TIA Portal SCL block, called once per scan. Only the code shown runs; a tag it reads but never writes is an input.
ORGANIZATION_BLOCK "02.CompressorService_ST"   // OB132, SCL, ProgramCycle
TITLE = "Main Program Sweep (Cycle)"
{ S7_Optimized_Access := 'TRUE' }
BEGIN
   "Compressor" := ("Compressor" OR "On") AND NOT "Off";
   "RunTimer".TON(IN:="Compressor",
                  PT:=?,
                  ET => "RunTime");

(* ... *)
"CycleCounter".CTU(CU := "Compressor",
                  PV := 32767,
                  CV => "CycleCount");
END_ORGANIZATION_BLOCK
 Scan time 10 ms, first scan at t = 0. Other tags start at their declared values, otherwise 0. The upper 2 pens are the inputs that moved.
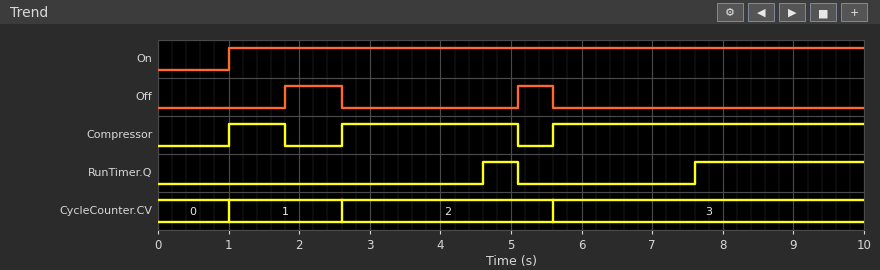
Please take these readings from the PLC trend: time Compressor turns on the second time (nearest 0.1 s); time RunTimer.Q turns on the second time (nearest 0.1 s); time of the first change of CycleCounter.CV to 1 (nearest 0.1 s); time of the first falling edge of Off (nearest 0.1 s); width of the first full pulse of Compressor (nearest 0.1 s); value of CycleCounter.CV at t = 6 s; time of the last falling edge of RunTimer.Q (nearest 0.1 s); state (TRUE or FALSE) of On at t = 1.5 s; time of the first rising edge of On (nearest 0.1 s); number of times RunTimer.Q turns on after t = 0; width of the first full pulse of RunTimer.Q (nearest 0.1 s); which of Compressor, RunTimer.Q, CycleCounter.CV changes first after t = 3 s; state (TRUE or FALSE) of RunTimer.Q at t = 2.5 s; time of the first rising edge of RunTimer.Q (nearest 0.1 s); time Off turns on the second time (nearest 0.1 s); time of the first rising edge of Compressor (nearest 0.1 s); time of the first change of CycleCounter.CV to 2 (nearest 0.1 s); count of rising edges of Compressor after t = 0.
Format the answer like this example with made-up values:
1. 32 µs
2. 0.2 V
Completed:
1. 2.6 s
2. 7.6 s
3. 1.0 s
4. 2.6 s
5. 0.8 s
6. 3
7. 5.1 s
8. TRUE
9. 1.0 s
10. 2
11. 0.5 s
12. RunTimer.Q
13. FALSE
14. 4.6 s
15. 5.1 s
16. 1.0 s
17. 2.6 s
18. 3
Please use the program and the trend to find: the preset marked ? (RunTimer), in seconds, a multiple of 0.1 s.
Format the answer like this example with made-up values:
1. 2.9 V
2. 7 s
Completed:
1. 2.0 s
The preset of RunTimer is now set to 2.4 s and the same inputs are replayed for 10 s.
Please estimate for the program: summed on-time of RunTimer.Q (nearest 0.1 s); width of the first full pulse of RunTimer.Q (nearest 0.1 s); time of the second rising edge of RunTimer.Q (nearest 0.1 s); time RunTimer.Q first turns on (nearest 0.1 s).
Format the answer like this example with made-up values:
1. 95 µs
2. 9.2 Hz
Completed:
1. 2.1 s
2. 0.1 s
3. 8.0 s
4. 5.0 s
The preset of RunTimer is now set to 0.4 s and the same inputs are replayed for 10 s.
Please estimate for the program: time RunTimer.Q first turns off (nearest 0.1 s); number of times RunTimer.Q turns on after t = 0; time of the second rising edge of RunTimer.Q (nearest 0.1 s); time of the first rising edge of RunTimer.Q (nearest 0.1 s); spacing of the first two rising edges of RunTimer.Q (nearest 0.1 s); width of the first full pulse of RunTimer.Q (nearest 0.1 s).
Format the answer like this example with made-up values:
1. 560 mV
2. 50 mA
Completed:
1. 1.8 s
2. 3
3. 3.0 s
4. 1.4 s
5. 1.6 s
6. 0.4 s
